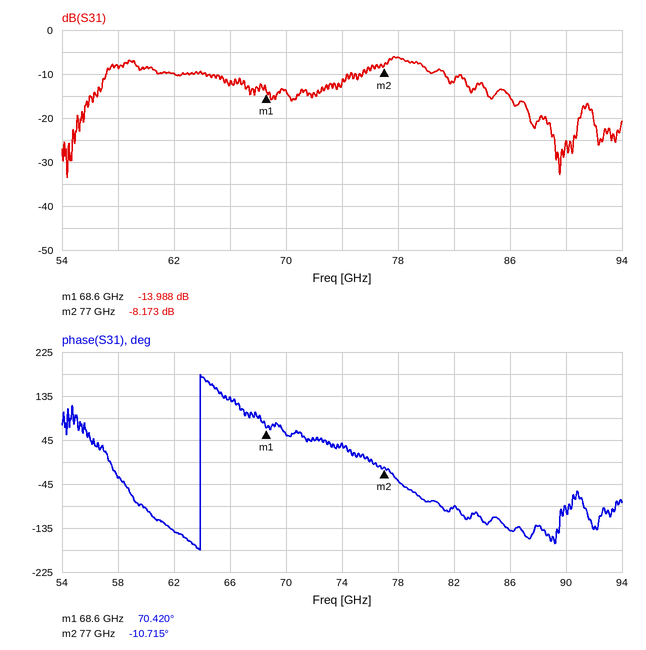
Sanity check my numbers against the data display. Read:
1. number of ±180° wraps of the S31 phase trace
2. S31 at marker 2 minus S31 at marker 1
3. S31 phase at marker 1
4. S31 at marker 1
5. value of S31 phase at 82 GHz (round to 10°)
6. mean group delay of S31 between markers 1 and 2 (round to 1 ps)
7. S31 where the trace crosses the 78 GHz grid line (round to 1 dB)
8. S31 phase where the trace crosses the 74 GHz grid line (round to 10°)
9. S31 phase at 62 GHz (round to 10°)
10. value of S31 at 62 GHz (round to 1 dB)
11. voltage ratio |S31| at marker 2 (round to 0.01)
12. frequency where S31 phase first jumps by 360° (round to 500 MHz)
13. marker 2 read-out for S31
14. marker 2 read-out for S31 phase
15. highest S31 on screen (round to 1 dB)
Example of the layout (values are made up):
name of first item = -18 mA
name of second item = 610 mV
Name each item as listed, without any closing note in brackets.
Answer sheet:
number of ±180° wraps of the S31 phase trace = 1
S31 at marker 2 minus S31 at marker 1 = 5.815 dB
S31 phase at marker 1 = 70.420°
S31 at marker 1 = -13.988 dB
value of S31 phase at 82 GHz = -90°
mean group delay of S31 between markers 1 and 2 = 27 ps
S31 where the trace crosses the 78 GHz grid line = -6 dB
S31 phase where the trace crosses the 74 GHz grid line = 40°
S31 phase at 62 GHz = -140°
value of S31 at 62 GHz = -10 dB
voltage ratio |S31| at marker 2 = 0.39
frequency where S31 phase first jumps by 360° = 64.0 GHz
marker 2 read-out for S31 = -8.173 dB
marker 2 read-out for S31 phase = -10.715°
highest S31 on screen = -6 dB
